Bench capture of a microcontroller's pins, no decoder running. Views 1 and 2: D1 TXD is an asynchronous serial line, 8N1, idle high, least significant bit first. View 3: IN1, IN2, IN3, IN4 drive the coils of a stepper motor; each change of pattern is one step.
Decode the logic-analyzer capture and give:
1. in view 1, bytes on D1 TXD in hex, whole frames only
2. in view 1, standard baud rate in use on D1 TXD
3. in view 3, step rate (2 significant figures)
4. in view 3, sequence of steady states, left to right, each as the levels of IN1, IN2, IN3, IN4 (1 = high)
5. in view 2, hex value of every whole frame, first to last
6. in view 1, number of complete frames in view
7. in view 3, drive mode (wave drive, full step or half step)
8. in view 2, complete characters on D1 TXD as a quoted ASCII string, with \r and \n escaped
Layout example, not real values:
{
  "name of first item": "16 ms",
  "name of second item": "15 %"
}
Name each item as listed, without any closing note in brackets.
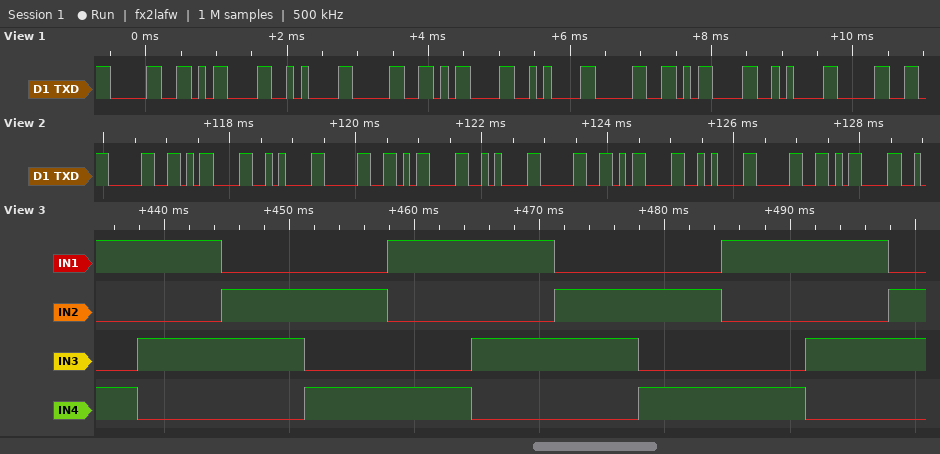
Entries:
{
  "in view 1, bytes on D1 TXD in hex, whole frames only": "30 0D 0A 30 0D 0A 30 0D 0A 30",
  "in view 1, standard baud rate in use on D1 TXD": "9600 baud",
  "in view 3, step rate": "150 steps/s",
  "in view 3, sequence of steady states, left to right, each as the levels of IN1, IN2, IN3, IN4": "1001 1010 0110 0101 1001 1010 0110 0101 1001 1010 0110",
  "in view 2, hex value of every whole frame, first to last": "30 0D 0A 30 0D 0A 30 0D 0A 30 0D",
  "in view 1, number of complete frames in view": "10",
  "in view 3, drive mode": "full step",
  "in view 2, complete characters on D1 TXD as a quoted ASCII string, with \\r and \\n escaped": "\"0\\r\\n0\\r\\n0\\r\\n0\\r\""
}
